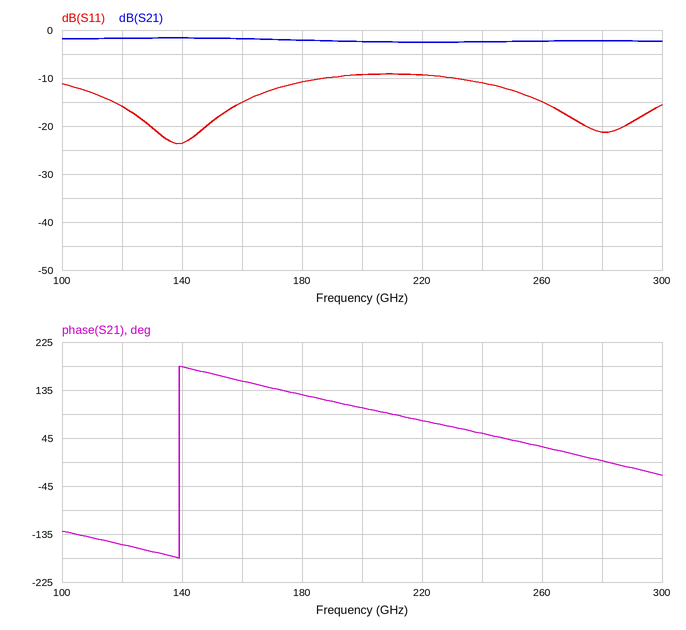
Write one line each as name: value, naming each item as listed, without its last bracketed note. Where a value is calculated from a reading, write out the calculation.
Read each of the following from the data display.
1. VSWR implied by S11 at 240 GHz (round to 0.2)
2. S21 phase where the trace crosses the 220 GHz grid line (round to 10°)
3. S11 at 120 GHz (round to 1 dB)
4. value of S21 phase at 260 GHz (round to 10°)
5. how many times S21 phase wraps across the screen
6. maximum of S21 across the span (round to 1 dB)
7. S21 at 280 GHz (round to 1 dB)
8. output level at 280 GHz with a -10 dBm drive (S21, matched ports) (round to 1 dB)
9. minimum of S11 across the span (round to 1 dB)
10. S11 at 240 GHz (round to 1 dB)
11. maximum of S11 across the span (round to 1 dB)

VSWR implied by S11 at 240 GHz: |Γ| = 10^(-11/20) = 0.2818; VSWR = (1 + 0.2818)/(1 − 0.2818) ≈ 1.8
S21 phase where the trace crosses the 220 GHz grid line: 80°
S11 at 120 GHz: -16 dB
value of S21 phase at 260 GHz: 30°
how many times S21 phase wraps across the screen: 1
maximum of S21 across the span: -2 dB
S21 at 280 GHz: -2 dB
output level at 280 GHz with a -10 dBm drive (S21, matched ports): -10 dBm + (-2 dB) = -12 dBm
minimum of S11 across the span: -24 dB
S11 at 240 GHz: -11 dB
maximum of S11 across the span: -9 dB
